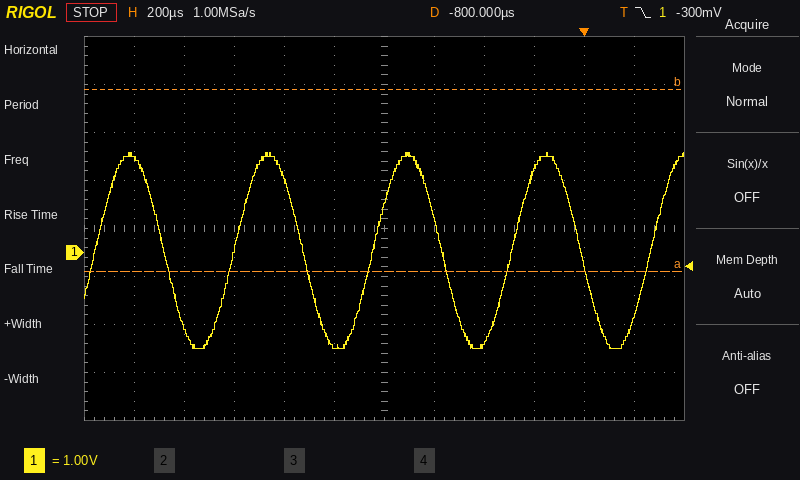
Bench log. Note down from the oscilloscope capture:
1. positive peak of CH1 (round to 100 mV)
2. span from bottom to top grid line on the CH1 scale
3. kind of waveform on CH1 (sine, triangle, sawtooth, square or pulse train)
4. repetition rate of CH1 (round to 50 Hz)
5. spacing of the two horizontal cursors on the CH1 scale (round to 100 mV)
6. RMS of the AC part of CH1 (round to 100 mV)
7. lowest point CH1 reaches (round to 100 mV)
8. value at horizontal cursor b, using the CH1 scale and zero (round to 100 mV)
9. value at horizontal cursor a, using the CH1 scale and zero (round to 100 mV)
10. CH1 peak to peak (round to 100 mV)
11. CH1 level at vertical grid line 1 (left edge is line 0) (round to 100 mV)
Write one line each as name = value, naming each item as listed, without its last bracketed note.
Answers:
positive peak of CH1 = 2.1 V
span from bottom to top grid line on the CH1 scale = 8 V
kind of waveform on CH1 = sine
repetition rate of CH1 = 1.80 kHz
spacing of the two horizontal cursors on the CH1 scale = 3.8 V
RMS of the AC part of CH1 = 1.4 V
lowest point CH1 reaches = -2.0 V
value at horizontal cursor b, using the CH1 scale and zero = 3.4 V
value at horizontal cursor a, using the CH1 scale and zero = -400 mV
CH1 peak to peak = 4.1 V
CH1 level at vertical grid line 1 (left edge is line 0) = 2.0 V
